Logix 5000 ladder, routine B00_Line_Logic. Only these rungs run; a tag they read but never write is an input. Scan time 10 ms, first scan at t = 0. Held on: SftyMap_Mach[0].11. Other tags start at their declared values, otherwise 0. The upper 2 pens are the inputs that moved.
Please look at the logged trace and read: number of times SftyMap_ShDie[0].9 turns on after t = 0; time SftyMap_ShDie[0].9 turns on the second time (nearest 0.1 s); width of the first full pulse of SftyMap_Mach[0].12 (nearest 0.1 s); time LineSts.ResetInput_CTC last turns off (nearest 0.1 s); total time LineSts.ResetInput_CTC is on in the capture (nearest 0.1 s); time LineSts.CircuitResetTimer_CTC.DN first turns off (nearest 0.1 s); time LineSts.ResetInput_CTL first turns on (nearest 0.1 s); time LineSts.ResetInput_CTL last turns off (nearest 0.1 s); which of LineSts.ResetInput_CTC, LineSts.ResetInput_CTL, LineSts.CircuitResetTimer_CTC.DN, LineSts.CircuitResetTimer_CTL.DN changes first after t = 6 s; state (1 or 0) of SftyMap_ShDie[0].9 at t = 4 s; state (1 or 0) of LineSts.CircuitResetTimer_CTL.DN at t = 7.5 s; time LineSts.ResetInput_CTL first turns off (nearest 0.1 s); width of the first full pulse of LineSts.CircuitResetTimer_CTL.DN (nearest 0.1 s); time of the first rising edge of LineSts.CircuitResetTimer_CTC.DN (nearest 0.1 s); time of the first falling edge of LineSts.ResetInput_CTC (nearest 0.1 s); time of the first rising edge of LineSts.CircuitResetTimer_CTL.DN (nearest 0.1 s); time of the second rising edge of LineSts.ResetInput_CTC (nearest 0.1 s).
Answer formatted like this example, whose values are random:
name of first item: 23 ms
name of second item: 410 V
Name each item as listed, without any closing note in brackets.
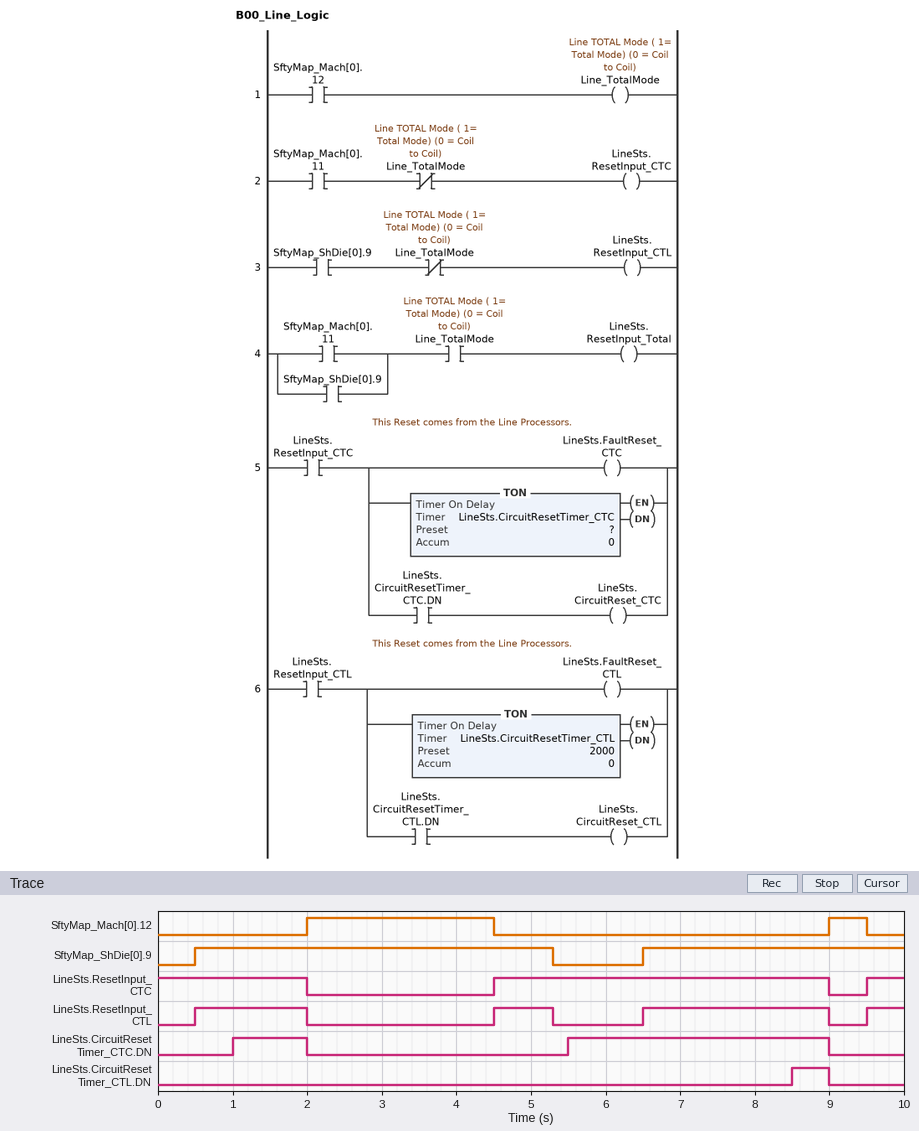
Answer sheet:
number of times SftyMap_ShDie[0].9 turns on after t = 0: 2
time SftyMap_ShDie[0].9 turns on the second time: 6.5 s
width of the first full pulse of SftyMap_Mach[0].12: 2.5 s
time LineSts.ResetInput_CTC last turns off: 9.0 s
total time LineSts.ResetInput_CTC is on in the capture: 7.0 s
time LineSts.CircuitResetTimer_CTC.DN first turns off: 2.0 s
time LineSts.ResetInput_CTL first turns on: 0.5 s
time LineSts.ResetInput_CTL last turns off: 9.0 s
which of LineSts.ResetInput_CTC, LineSts.ResetInput_CTL, LineSts.CircuitResetTimer_CTC.DN, LineSts.CircuitResetTimer_CTL.DN changes first after t = 6 s: LineSts.ResetInput_CTL
state (1 or 0) of SftyMap_ShDie[0].9 at t = 4 s: 1
state (1 or 0) of LineSts.CircuitResetTimer_CTL.DN at t = 7.5 s: 0
time LineSts.ResetInput_CTL first turns off: 2.0 s
width of the first full pulse of LineSts.CircuitResetTimer_CTL.DN: 0.5 s
time of the first rising edge of LineSts.CircuitResetTimer_CTC.DN: 1.0 s
time of the first falling edge of LineSts.ResetInput_CTC: 2.0 s
time of the first rising edge of LineSts.CircuitResetTimer_CTL.DN: 8.5 s
time of the second rising edge of LineSts.ResetInput_CTC: 9.5 s
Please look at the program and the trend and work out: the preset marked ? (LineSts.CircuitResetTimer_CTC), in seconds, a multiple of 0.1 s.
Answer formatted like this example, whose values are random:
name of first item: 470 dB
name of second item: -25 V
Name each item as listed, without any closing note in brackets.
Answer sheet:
the preset marked ? (LineSts.CircuitResetTimer_CTC), in seconds, a multiple of 0.1 s: 1.0 s
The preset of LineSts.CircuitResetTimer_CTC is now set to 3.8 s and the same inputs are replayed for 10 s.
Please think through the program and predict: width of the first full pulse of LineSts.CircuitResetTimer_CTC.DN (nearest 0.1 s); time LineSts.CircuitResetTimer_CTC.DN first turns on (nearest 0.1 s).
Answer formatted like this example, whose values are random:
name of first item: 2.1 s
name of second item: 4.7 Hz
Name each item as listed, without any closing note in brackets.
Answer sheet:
width of the first full pulse of LineSts.CircuitResetTimer_CTC.DN: 0.7 s
time LineSts.CircuitResetTimer_CTC.DN first turns on: 8.3 s
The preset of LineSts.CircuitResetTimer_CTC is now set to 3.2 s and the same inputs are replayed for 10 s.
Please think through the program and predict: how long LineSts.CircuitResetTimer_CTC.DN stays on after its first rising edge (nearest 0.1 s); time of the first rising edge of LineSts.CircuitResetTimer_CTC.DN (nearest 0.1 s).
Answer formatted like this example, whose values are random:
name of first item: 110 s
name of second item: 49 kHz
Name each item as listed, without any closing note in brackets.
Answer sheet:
how long LineSts.CircuitResetTimer_CTC.DN stays on after its first rising edge: 1.3 s
time of the first rising edge of LineSts.CircuitResetTimer_CTC.DN: 7.7 s
